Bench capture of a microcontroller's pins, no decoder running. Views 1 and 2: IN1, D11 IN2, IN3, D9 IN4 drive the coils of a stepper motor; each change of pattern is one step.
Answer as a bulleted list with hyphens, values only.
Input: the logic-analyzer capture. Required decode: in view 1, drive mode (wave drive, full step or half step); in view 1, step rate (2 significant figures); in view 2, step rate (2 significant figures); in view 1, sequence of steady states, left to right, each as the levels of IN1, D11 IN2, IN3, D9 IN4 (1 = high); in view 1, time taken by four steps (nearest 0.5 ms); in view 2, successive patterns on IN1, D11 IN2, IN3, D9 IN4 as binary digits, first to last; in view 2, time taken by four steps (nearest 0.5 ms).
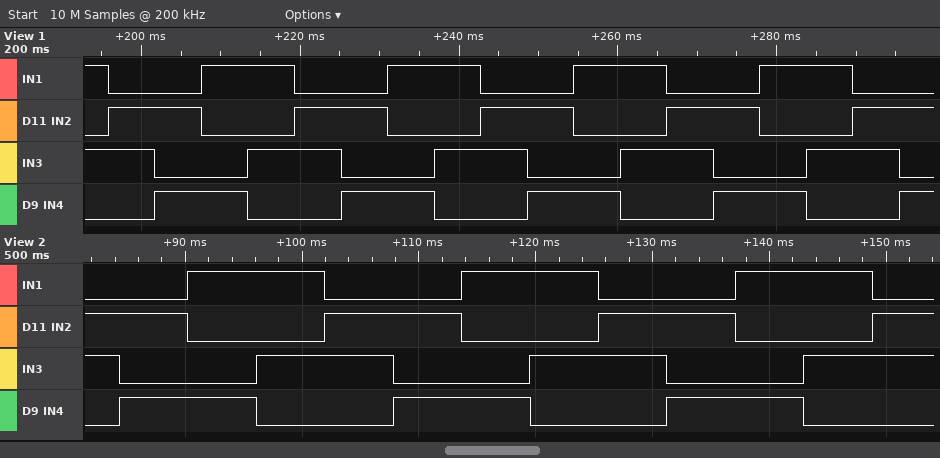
- full step
- 170 steps/s
- 170 steps/s
- 1010 0110 0101 1001 1010 0110 0101 1001 1010 0110 0101 1001 1010 0110 0101 1001 1010 0110 0101
- 23.5 ms
- 0110 0101 1001 1010 0110 0101 1001 1010 0110 0101 1001 1010 0110
- 23.5 ms
